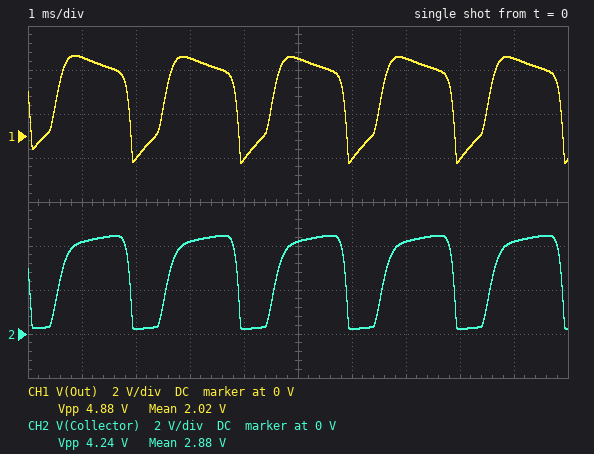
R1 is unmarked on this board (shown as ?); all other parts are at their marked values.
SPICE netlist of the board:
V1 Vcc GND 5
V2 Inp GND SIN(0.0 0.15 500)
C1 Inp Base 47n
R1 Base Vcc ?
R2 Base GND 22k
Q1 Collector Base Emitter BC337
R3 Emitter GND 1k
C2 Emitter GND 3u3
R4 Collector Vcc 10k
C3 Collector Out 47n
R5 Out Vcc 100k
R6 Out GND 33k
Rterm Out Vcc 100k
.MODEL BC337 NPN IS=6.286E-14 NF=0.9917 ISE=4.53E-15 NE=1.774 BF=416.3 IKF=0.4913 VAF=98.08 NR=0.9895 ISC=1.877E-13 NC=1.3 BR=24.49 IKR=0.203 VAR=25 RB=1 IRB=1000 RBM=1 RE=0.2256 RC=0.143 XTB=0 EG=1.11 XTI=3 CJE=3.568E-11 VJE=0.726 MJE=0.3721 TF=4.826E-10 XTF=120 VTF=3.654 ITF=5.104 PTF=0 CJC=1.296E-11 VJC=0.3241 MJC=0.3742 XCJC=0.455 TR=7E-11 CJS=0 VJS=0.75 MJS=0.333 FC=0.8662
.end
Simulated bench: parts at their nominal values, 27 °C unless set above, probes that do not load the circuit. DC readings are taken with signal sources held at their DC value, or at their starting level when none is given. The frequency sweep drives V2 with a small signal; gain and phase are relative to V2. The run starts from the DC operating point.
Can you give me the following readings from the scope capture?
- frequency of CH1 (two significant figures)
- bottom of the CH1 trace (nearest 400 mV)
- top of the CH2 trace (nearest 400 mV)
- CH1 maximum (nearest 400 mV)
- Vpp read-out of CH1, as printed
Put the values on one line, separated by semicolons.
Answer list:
500 Hz; -1.2 V; 4.4 V; 3.6 V; 4.88 V
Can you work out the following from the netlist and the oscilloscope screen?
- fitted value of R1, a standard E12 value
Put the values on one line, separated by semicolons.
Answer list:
120 kΩ
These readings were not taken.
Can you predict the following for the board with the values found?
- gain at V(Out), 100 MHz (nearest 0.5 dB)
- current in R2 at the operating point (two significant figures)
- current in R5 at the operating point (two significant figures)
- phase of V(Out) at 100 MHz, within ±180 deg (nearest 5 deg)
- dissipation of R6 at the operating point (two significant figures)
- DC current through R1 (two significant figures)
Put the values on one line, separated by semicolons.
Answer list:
7.5 dB; 35 µA; 30 µA; 65 deg; 120 µW; 35 µA
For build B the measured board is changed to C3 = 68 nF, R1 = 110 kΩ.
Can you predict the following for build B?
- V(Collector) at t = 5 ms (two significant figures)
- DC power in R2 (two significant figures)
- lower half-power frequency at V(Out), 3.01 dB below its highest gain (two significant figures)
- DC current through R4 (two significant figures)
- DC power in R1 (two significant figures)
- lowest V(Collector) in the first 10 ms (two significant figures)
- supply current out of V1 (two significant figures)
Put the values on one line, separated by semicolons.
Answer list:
4.1 V; 31 µW; 660 Hz; 250 µA; 160 µW; 250 mV; 350 µA
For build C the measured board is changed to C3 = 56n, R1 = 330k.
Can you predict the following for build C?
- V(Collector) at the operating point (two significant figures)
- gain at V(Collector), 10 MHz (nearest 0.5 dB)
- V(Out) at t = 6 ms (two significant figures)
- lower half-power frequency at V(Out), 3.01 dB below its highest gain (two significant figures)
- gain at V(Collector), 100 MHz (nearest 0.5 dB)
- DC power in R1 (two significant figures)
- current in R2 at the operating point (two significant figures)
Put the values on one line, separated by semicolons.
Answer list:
5.0 V; -1.0 dB; 2.0 V; 5.1 MHz; 0 dB; 67 µW; 14 µA
